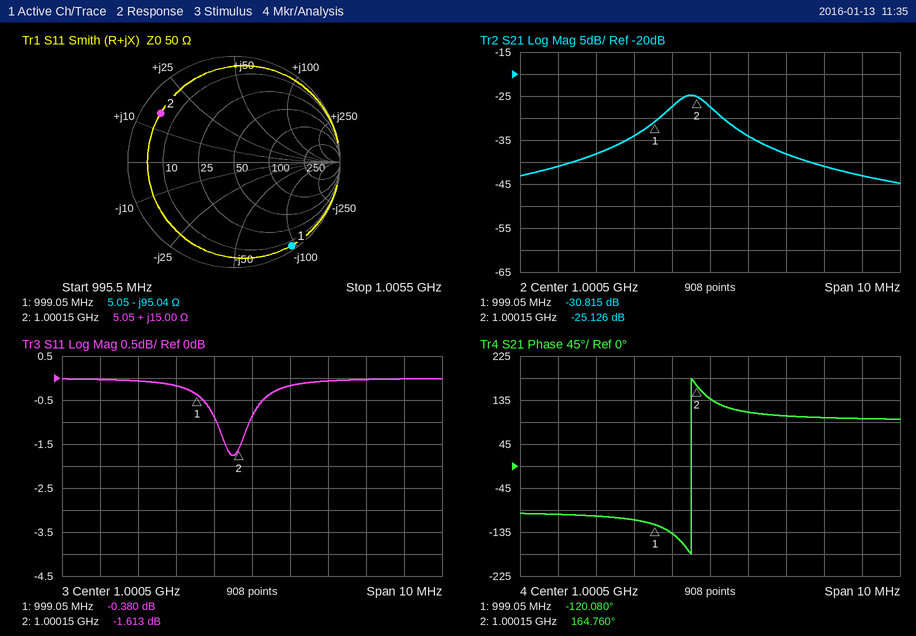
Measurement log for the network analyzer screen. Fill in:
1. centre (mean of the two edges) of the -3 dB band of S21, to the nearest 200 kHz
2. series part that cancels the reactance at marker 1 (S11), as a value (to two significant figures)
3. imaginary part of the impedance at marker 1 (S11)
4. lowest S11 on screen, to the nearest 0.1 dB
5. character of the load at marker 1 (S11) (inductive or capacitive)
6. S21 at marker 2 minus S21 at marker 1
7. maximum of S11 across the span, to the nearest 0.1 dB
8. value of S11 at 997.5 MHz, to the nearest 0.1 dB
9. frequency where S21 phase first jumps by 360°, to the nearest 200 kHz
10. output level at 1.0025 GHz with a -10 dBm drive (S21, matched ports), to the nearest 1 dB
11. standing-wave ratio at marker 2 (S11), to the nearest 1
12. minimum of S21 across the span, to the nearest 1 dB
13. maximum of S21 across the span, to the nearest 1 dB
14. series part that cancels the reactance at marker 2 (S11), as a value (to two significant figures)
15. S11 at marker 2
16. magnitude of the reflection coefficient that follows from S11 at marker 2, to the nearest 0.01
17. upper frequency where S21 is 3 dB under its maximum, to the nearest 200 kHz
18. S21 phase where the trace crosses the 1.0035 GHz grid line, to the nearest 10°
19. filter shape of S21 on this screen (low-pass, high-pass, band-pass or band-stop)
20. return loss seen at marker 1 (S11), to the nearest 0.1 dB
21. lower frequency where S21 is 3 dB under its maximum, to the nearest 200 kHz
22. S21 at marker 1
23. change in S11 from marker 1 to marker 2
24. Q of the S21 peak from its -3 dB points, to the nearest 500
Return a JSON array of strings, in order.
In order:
["1.0000 GHz", "15 nH", "-95.04 Ω", "-1.8 dB", "capacitive", "5.689 dB", "0.0 dB", "-0.1 dB", "1.0000 GHz", "-48 dBm", "11", "-45 dB", "-25 dB", "11 pF", "-1.613 dB", "0.83", "1.0006 GHz", "100°", "band-pass", "0.4 dB", "999.4 MHz", "-30.815 dB", "-1.233 dB", "1000"]
